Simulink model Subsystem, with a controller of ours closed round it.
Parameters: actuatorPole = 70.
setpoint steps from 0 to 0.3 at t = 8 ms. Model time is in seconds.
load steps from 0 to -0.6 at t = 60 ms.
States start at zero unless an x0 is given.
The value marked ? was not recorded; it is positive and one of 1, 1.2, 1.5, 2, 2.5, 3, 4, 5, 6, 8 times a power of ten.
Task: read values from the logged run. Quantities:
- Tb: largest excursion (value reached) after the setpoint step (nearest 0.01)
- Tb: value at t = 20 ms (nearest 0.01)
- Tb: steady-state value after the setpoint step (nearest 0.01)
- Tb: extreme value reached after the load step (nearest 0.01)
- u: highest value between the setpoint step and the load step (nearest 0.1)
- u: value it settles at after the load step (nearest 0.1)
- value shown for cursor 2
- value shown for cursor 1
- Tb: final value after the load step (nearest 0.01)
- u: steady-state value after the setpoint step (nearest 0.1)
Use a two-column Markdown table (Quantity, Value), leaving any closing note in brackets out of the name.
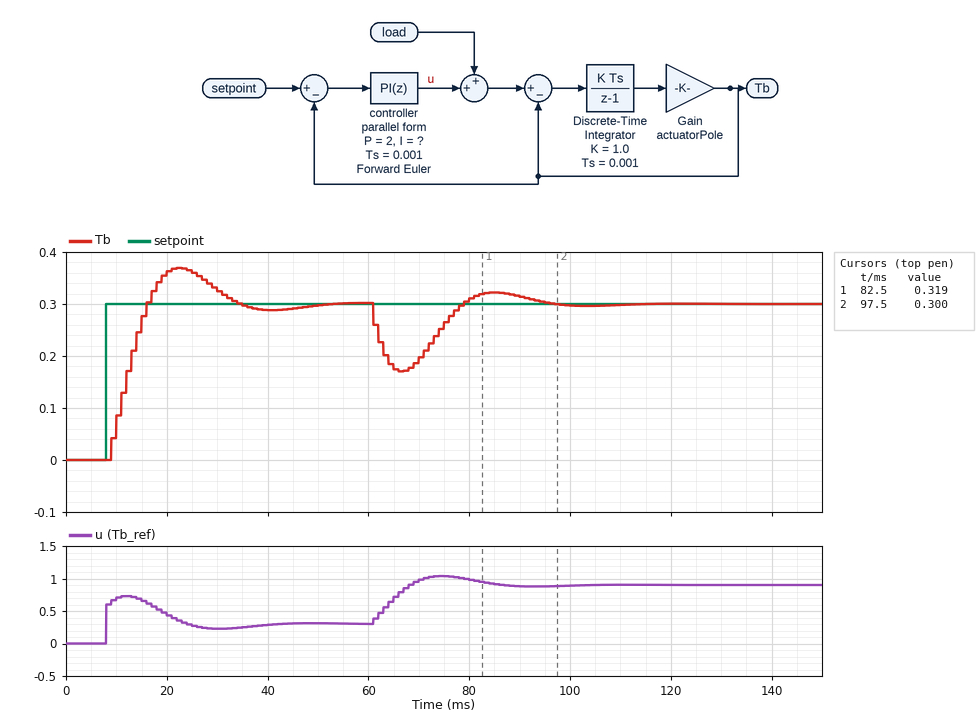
| Quantity | Value |
|---|---|
| Tb: largest excursion (value reached) after the setpoint step | 0.37 |
| Tb: value at t = 20 ms | 0.36 |
| Tb: steady-state value after the setpoint step | 0.30 |
| Tb: extreme value reached after the load step | 0.17 |
| u: highest value between the setpoint step and the load step | 0.7 |
| u: value it settles at after the load step | 0.9 |
| value shown for cursor 2 | 0.300 |
| value shown for cursor 1 | 0.319 |
| Tb: final value after the load step | 0.30 |
| u: steady-state value after the setpoint step | 0.3 |
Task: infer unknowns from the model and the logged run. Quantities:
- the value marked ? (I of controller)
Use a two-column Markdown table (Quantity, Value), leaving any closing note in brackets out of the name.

| Quantity | Value |
|---|---|
| the value marked ? | 500 |
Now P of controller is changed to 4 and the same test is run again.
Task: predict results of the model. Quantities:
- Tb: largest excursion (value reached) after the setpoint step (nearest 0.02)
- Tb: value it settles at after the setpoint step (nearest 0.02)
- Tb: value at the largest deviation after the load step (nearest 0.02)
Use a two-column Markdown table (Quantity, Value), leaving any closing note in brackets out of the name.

| Quantity | Value |
|---|---|
| Tb: largest excursion (value reached) after the setpoint step | 0.32 |
| Tb: value it settles at after the setpoint step | 0.30 |
| Tb: value at the largest deviation after the load step | 0.20 |
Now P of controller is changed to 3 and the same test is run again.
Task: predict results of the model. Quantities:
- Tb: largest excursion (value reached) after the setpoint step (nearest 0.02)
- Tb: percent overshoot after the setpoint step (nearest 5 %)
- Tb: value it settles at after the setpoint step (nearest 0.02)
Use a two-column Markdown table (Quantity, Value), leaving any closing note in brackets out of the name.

| Quantity | Value |
|---|---|
| Tb: largest excursion (value reached) after the setpoint step | 0.34 |
| Tb: percent overshoot after the setpoint step | 15 % |
| Tb: value it settles at after the setpoint step | 0.30 |
